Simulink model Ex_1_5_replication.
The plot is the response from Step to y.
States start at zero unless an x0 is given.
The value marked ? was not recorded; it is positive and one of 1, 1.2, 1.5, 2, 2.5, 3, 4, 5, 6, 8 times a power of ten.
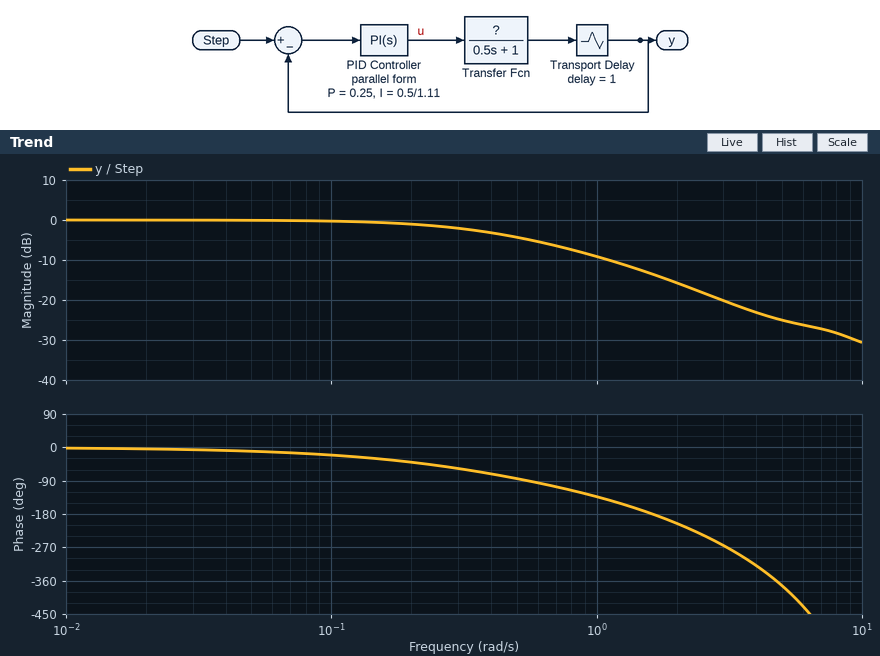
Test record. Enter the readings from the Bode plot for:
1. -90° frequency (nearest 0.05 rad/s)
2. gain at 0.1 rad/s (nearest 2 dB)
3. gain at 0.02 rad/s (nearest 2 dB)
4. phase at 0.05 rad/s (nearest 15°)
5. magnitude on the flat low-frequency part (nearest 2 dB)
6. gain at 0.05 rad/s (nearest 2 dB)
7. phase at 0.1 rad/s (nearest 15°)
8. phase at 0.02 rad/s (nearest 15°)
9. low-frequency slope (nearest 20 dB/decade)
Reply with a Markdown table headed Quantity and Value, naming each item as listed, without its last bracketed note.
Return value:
| Quantity | Value |
|---|---|
| -90° frequency | 0.55 rad/s |
| gain at 0.1 rad/s | 0 dB |
| gain at 0.02 rad/s | 0 dB |
| phase at 0.05 rad/s | -15° |
| magnitude on the flat low-frequency part | 0 dB |
| gain at 0.05 rad/s | 0 dB |
| phase at 0.1 rad/s | -15° |
| phase at 0.02 rad/s | 0° |
| low-frequency slope | 0 dB/decade |
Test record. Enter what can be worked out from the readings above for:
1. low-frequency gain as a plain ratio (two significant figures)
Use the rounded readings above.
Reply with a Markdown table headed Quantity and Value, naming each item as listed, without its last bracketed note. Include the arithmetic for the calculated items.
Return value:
| Quantity | Value |
|---|---|
| low-frequency gain as a plain ratio | 10^(0 / 20) = 1.0 |
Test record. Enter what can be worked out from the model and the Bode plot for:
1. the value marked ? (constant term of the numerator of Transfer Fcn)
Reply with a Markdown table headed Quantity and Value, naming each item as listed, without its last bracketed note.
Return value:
| Quantity | Value |
|---|---|
| the value marked ? | 0.6 |
